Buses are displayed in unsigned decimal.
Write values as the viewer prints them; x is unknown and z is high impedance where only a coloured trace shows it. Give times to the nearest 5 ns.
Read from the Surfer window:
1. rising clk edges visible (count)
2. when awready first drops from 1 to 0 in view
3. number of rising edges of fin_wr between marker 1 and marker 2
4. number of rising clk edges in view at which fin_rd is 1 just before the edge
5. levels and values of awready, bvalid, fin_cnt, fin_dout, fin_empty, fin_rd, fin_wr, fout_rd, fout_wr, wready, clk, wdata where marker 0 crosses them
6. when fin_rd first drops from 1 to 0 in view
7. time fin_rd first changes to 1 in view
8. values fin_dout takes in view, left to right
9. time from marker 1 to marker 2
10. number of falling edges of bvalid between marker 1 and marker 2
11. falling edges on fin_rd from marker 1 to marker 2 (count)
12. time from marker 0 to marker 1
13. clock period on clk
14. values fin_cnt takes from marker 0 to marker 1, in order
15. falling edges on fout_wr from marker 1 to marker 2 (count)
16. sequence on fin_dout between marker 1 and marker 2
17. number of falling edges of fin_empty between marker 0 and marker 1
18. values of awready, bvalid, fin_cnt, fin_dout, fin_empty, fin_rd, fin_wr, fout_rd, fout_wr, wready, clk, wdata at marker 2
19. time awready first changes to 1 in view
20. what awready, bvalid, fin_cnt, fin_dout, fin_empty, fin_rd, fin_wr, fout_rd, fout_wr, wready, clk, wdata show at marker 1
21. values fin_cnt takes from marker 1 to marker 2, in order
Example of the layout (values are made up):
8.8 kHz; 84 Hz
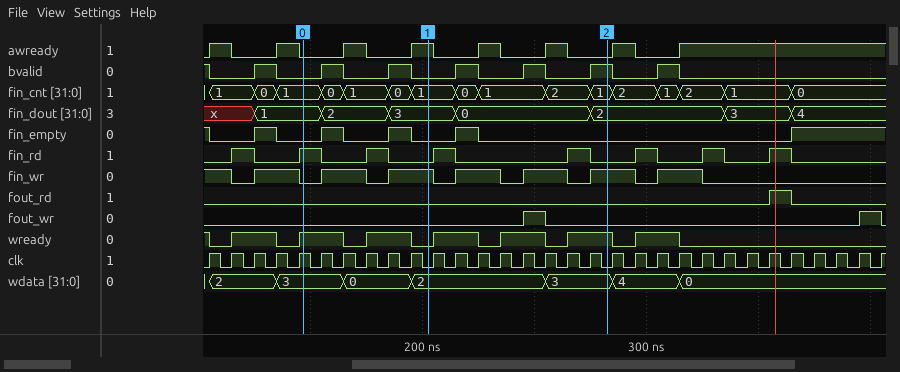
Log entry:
31; 115 ns; 3; 8; awready=0, bvalid=0, fin_cnt=1, fin_dout=1, fin_empty=0, fin_rd=1, fin_wr=0, fout_rd=0, fout_wr=0, wready=1, clk=1, wdata=3; 125 ns; 115 ns; x, 1, 2, 3, 0, 2, 3, 4; 80 ns; 2; 2; 55 ns; 10 ns; 1, 0, 1, 0, 1; 1; 3, 0, 2; 2; awready=0, bvalid=1, fin_cnt=1, fin_dout=2, fin_empty=0, fin_rd=0, fin_wr=1, fout_rd=0, fout_wr=0, wready=1, clk=0, wdata=3; 105 ns; awready=1, bvalid=0, fin_cnt=1, fin_dout=3, fin_empty=0, fin_rd=0, fin_wr=1, fout_rd=0, fout_wr=0, wready=0, clk=0, wdata=2; 1, 0, 1, 2, 1
